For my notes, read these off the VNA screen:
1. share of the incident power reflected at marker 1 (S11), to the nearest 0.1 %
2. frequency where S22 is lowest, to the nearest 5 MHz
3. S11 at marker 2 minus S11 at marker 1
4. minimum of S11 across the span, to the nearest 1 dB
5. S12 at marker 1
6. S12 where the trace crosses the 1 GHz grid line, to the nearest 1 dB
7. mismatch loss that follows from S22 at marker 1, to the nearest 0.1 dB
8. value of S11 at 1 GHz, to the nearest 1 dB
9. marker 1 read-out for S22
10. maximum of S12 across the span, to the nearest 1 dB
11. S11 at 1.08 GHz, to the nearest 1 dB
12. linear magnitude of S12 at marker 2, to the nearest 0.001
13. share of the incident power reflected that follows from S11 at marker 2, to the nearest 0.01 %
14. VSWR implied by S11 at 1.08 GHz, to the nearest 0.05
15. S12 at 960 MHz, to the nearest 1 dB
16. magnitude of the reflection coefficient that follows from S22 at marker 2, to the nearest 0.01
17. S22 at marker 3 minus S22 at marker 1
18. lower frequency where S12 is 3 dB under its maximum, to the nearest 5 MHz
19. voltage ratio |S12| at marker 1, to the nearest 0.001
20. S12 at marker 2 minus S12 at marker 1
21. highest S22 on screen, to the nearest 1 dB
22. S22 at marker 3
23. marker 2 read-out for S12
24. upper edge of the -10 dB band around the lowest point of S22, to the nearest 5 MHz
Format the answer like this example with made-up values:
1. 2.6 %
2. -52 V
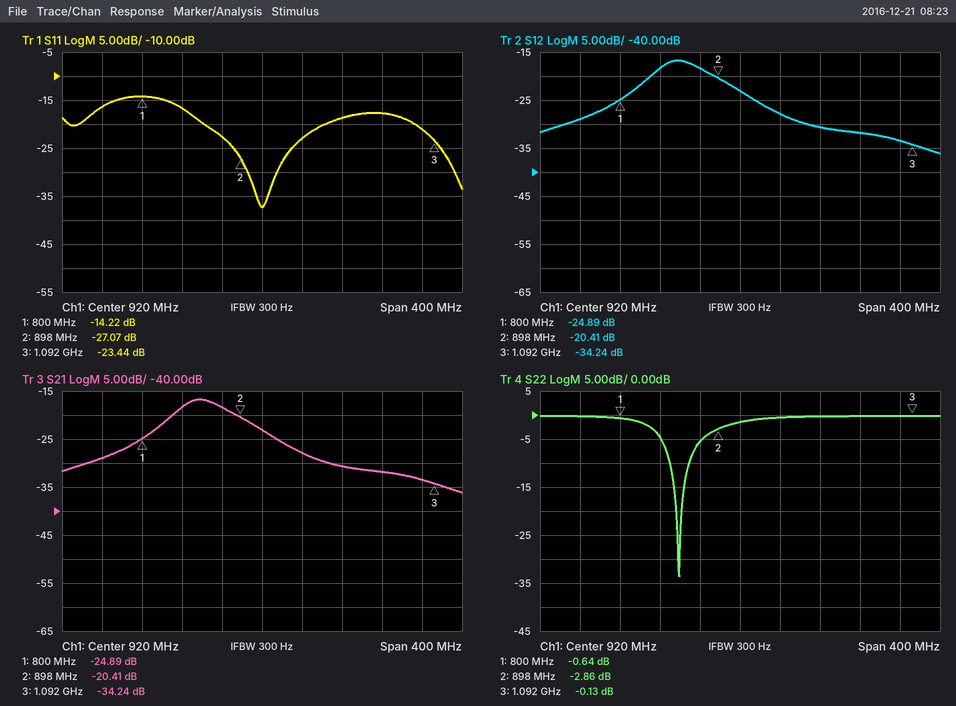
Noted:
1. 3.8 %
2. 860 MHz
3. -12.85 dB
4. -37 dB
5. -24.89 dB
6. -31 dB
7. 8.6 dB
8. -19 dB
9. -0.64 dB
10. -17 dB
11. -21 dB
12. 0.095
13. 0.20 %
14. 1.20
15. -28 dB
16. 0.72
17. 0.51 dB
18. 830 MHz
19. 0.057
20. 4.48 dB
21. 0 dB
22. -0.13 dB
23. -20.41 dB
24. 870 MHz
